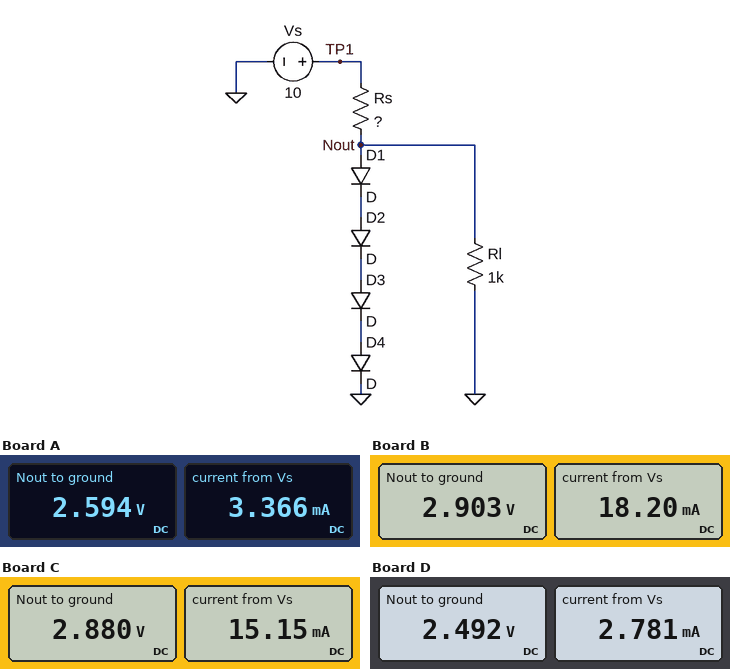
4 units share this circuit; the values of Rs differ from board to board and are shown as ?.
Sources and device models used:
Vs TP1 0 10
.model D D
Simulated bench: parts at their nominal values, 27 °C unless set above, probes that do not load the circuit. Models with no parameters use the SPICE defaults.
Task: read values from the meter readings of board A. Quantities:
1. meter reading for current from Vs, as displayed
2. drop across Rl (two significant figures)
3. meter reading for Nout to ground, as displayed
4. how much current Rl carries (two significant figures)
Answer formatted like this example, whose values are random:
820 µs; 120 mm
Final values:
3.366 mA; 2.6 V; 2.594 V; 2.6 mA
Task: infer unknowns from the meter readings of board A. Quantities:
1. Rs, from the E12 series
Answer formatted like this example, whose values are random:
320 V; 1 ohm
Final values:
2.2 kΩ
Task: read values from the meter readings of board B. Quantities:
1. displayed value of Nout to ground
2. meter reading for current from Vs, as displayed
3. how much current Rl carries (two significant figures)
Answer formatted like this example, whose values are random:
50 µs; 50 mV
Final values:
2.903 V; 18.20 mA; 2.9 mA
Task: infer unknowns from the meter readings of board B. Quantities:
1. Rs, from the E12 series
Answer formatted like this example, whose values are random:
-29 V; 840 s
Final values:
390 Ω
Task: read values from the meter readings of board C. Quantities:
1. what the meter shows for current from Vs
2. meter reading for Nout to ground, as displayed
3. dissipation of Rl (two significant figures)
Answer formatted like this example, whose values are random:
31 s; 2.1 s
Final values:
15.15 mA; 2.880 V; 8.3 mW
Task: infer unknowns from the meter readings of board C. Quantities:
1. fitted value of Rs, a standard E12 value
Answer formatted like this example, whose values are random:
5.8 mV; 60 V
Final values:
470 Ω
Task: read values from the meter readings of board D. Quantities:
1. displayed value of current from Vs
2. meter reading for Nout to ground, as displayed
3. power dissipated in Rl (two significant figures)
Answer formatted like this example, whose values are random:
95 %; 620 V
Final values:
2.781 mA; 2.492 V; 6.2 mW
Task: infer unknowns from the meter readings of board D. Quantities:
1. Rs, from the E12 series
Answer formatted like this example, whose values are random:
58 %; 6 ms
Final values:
2.7 kΩ
